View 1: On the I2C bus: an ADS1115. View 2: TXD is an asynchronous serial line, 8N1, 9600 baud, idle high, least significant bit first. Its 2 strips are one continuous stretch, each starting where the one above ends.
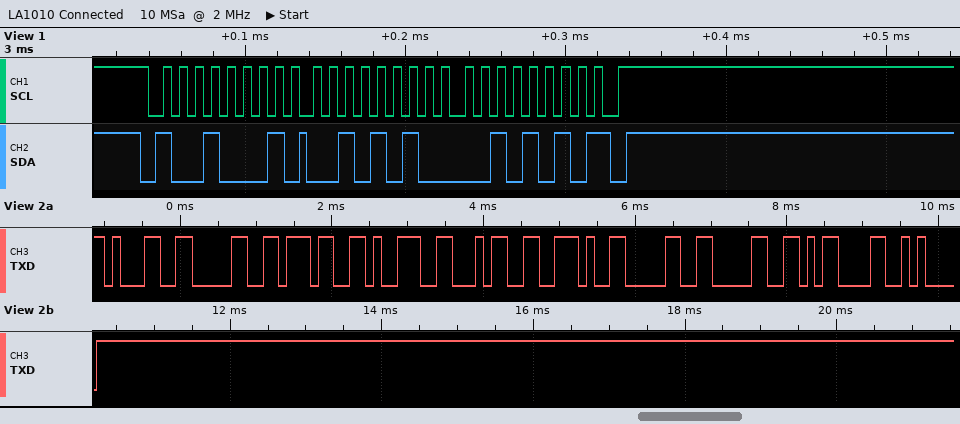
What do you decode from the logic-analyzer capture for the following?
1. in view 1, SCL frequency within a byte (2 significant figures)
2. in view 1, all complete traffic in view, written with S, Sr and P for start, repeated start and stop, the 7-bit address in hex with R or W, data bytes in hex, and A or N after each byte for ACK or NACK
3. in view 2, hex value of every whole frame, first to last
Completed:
100 kHz
S 48R A 2A A 2A N P
31 30 37 39 34 2E 30 30 0D 0A
